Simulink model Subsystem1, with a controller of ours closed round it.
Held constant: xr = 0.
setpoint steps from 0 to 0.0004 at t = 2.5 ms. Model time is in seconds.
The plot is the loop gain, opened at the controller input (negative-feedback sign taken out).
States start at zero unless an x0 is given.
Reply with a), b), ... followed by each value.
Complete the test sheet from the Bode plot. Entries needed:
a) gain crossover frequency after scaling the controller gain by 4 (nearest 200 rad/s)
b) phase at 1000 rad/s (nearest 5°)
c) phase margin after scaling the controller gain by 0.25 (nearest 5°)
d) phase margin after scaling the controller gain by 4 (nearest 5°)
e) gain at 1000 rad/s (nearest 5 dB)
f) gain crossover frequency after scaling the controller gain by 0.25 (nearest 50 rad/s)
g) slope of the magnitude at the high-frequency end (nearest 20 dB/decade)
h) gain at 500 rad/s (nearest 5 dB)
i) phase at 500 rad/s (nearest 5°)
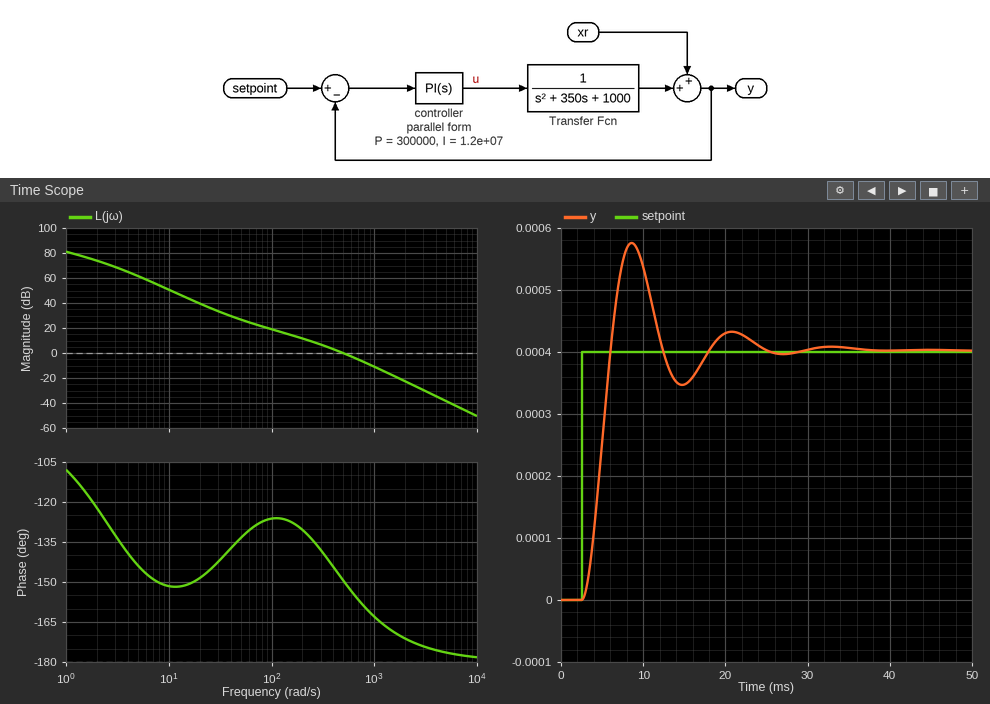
a) 1000 rad/s
b) -165°
c) 50°
d) 15°
e) -10 dB
f) 200 rad/s
g) -40 dB/decade
h) 0 dB
i) -150°
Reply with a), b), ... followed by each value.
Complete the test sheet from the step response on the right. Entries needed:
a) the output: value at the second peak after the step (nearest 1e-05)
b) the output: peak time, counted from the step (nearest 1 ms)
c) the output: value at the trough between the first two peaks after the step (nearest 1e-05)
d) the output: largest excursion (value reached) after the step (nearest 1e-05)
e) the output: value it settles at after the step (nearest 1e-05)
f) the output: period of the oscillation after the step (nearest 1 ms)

a) 0.00043
b) 6 ms
c) 0.00035
d) 0.00058
e) 0.00040
f) 12 ms
